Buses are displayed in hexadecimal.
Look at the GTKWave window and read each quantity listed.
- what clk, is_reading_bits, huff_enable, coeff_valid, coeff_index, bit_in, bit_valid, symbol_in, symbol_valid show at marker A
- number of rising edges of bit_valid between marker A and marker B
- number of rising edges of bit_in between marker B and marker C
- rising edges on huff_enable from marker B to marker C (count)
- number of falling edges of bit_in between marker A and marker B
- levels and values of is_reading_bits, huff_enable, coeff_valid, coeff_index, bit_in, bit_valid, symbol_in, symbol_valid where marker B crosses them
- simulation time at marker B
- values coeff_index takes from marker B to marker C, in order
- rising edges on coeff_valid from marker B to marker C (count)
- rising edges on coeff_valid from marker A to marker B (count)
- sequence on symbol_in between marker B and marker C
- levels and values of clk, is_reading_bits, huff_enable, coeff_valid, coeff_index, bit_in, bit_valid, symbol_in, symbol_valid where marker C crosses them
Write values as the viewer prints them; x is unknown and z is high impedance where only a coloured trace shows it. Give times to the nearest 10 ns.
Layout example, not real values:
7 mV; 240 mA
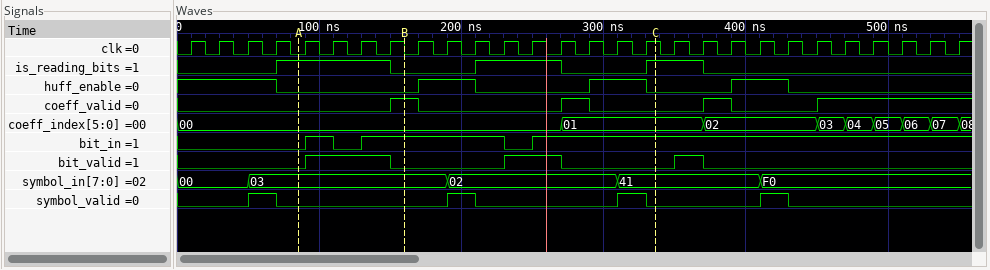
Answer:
clk=0, is_reading_bits=1, huff_enable=0, coeff_valid=0, coeff_index=00, bit_in=0, bit_valid=0, symbol_in=03, symbol_valid=0; 1; 1; 2; 1; is_reading_bits=0, huff_enable=0, coeff_valid=1, coeff_index=00, bit_in=1, bit_valid=0, symbol_in=03, symbol_valid=0; 160 ns; 00, 01; 1; 1; 03, 02, 41; clk=1, is_reading_bits=1, huff_enable=0, coeff_valid=0, coeff_index=01, bit_in=1, bit_valid=0, symbol_in=41, symbol_valid=0
